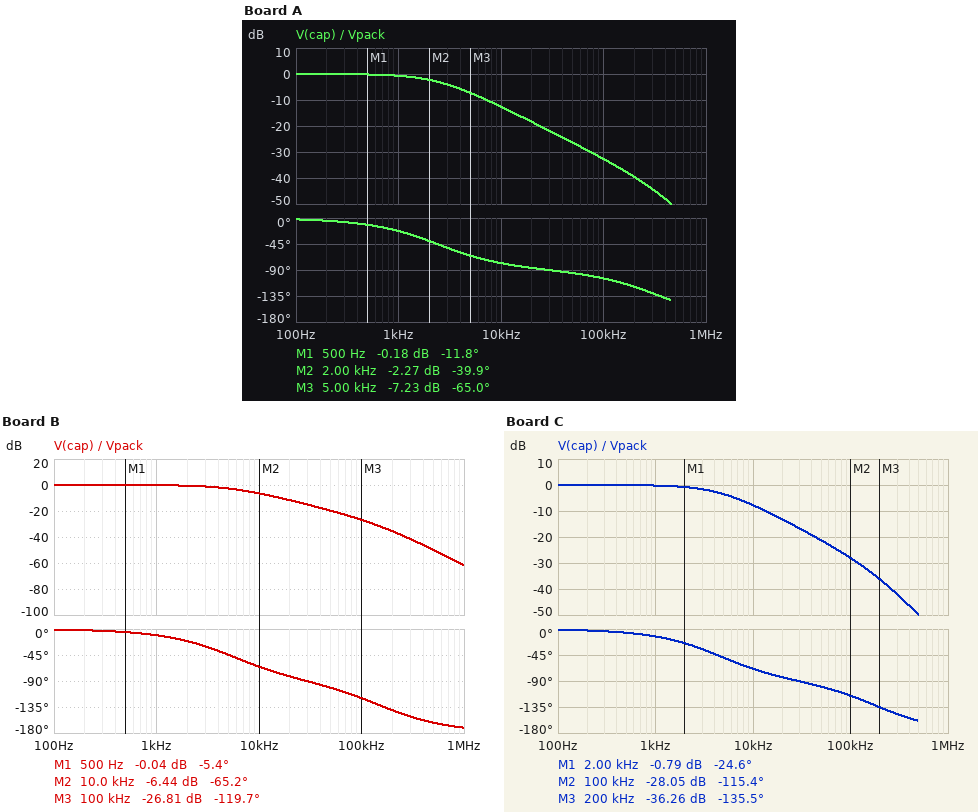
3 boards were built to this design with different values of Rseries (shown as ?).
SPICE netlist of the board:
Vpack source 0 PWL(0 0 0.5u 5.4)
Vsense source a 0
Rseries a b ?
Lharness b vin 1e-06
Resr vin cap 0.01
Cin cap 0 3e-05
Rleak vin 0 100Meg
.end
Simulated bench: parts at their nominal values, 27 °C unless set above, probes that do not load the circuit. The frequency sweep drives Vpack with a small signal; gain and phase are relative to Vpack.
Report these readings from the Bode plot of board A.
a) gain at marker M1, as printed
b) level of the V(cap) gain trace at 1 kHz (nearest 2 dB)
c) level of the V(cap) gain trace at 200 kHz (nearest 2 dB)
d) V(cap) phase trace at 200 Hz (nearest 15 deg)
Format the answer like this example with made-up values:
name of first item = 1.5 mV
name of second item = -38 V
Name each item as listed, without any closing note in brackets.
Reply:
gain at marker M1, as printed = -0.18 dB
level of the V(cap) gain trace at 1 kHz = 0 dB
level of the V(cap) gain trace at 200 kHz = -40 dB
V(cap) phase trace at 200 Hz = 0 deg
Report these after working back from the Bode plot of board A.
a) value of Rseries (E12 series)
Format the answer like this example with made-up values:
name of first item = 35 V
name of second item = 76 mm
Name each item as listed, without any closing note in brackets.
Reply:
value of Rseries = 2.2 Ω
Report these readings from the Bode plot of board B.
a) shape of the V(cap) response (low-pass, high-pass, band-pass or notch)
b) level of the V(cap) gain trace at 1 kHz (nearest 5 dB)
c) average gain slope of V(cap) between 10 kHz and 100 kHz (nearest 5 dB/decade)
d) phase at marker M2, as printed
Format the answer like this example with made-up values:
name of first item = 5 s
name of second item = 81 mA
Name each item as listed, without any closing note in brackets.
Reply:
shape of the V(cap) response = low-pass
level of the V(cap) gain trace at 1 kHz = 0 dB
average gain slope of V(cap) between 10 kHz and 100 kHz = -20 dB/decade
phase at marker M2, as printed = -65.2 deg
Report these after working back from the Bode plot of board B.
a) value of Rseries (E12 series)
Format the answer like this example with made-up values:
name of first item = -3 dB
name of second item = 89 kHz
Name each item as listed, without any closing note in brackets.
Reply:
value of Rseries = 1 Ω
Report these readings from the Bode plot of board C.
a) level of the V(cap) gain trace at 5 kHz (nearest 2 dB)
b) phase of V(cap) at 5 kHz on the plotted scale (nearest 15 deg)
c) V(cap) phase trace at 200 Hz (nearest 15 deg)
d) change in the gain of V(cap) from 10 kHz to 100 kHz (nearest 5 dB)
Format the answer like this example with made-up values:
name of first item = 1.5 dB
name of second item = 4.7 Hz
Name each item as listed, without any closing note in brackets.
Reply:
level of the V(cap) gain trace at 5 kHz = -4 dB
phase of V(cap) at 5 kHz on the plotted scale = -45 deg
V(cap) phase trace at 200 Hz = 0 deg
change in the gain of V(cap) from 10 kHz to 100 kHz = -20 dB
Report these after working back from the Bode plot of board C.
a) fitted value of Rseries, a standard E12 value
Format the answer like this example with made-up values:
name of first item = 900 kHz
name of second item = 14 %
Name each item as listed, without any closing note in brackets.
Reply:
fitted value of Rseries, a standard E12 value = 1.2 Ω
